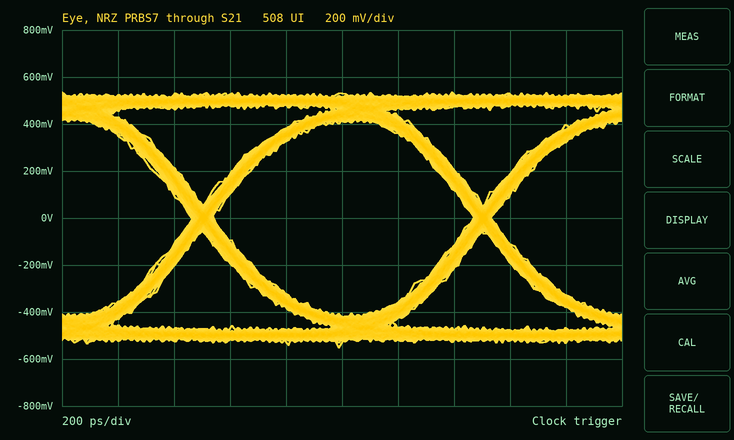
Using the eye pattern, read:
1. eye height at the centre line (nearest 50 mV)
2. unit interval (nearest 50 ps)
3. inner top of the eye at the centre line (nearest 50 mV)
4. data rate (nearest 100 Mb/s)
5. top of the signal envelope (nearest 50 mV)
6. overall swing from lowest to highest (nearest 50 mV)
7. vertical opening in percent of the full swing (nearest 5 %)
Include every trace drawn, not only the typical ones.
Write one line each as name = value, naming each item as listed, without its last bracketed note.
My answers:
eye height at the centre line = 850 mV
unit interval = 1.00 ns
inner top of the eye at the centre line = 400 mV
data rate = 1.0 Gb/s
top of the signal envelope = 550 mV
overall swing from lowest to highest = 1.10 V
vertical opening in percent of the full swing = 75 %
